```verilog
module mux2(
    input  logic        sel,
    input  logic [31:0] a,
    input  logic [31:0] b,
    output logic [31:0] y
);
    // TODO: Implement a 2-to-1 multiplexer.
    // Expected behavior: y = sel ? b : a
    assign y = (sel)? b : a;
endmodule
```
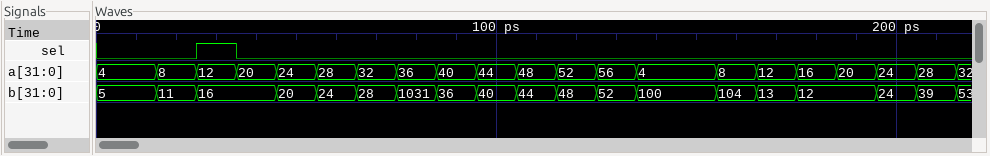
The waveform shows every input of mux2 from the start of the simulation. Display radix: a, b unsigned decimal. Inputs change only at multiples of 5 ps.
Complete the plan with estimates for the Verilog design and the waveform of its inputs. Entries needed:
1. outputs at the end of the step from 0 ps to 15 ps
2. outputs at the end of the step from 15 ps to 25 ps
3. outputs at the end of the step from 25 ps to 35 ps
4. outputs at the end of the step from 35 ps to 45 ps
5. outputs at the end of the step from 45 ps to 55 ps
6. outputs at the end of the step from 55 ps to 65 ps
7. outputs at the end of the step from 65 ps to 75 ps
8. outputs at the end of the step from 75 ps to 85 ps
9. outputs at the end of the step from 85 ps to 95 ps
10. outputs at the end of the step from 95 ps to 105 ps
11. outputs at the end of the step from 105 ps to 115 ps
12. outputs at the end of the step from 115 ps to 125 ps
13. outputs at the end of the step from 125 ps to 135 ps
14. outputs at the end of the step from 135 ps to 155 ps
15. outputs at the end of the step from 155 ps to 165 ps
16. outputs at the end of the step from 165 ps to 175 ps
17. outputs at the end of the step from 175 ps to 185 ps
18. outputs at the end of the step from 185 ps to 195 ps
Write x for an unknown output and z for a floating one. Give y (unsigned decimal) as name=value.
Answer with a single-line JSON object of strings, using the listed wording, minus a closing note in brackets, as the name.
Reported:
{"outputs at the end of the step from 0 ps to 15 ps": "y=4", "outputs at the end of the step from 15 ps to 25 ps": "y=8", "outputs at the end of the step from 25 ps to 35 ps": "y=16", "outputs at the end of the step from 35 ps to 45 ps": "y=20", "outputs at the end of the step from 45 ps to 55 ps": "y=24", "outputs at the end of the step from 55 ps to 65 ps": "y=28", "outputs at the end of the step from 65 ps to 75 ps": "y=32", "outputs at the end of the step from 75 ps to 85 ps": "y=36", "outputs at the end of the step from 85 ps to 95 ps": "y=40", "outputs at the end of the step from 95 ps to 105 ps": "y=44", "outputs at the end of the step from 105 ps to 115 ps": "y=48", "outputs at the end of the step from 115 ps to 125 ps": "y=52", "outputs at the end of the step from 125 ps to 135 ps": "y=56", "outputs at the end of the step from 135 ps to 155 ps": "y=4", "outputs at the end of the step from 155 ps to 165 ps": "y=8", "outputs at the end of the step from 165 ps to 175 ps": "y=12", "outputs at the end of the step from 175 ps to 185 ps": "y=16", "outputs at the end of the step from 185 ps to 195 ps": "y=20"}
